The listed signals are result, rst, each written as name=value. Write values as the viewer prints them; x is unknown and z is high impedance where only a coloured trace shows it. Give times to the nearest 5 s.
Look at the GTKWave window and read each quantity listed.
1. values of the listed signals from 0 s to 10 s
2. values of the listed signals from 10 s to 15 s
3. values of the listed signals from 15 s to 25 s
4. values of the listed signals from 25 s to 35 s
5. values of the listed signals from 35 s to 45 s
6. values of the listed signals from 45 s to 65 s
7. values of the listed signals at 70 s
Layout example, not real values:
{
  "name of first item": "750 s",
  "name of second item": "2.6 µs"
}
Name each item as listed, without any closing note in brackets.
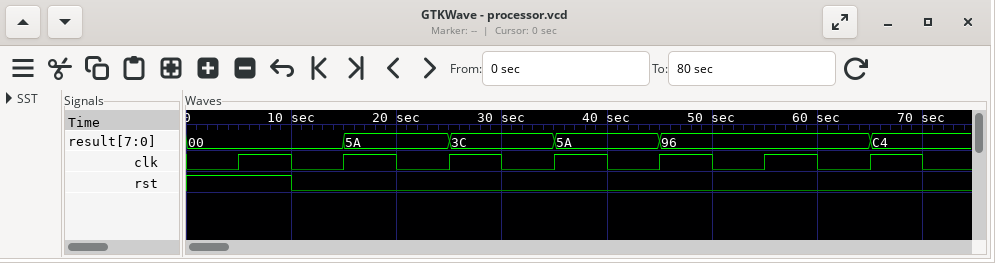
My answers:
{
  "values of the listed signals from 0 s to 10 s": "result=00, rst=1",
  "values of the listed signals from 10 s to 15 s": "result=00, rst=0",
  "values of the listed signals from 15 s to 25 s": "result=5A, rst=0",
  "values of the listed signals from 25 s to 35 s": "result=3C, rst=0",
  "values of the listed signals from 35 s to 45 s": "result=5A, rst=0",
  "values of the listed signals from 45 s to 65 s": "result=96, rst=0",
  "values of the listed signals at 70 s": "result=C4, rst=0"
}
